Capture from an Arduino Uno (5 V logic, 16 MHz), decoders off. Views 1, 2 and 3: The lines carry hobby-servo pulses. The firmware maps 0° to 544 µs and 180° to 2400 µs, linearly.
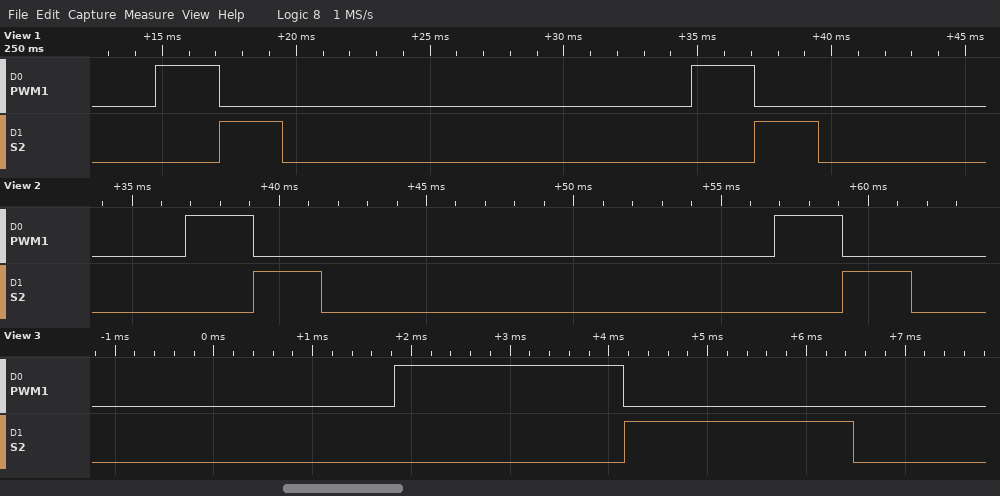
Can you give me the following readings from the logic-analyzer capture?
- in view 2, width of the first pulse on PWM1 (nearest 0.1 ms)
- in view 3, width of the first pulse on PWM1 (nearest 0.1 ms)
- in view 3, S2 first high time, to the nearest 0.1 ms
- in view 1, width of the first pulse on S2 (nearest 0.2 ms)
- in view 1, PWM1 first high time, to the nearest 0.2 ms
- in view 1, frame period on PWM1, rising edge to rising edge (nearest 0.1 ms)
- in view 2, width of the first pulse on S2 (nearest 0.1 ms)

2.3 ms
2.3 ms
2.3 ms
2.4 ms
2.4 ms
20.0 ms
2.3 ms
